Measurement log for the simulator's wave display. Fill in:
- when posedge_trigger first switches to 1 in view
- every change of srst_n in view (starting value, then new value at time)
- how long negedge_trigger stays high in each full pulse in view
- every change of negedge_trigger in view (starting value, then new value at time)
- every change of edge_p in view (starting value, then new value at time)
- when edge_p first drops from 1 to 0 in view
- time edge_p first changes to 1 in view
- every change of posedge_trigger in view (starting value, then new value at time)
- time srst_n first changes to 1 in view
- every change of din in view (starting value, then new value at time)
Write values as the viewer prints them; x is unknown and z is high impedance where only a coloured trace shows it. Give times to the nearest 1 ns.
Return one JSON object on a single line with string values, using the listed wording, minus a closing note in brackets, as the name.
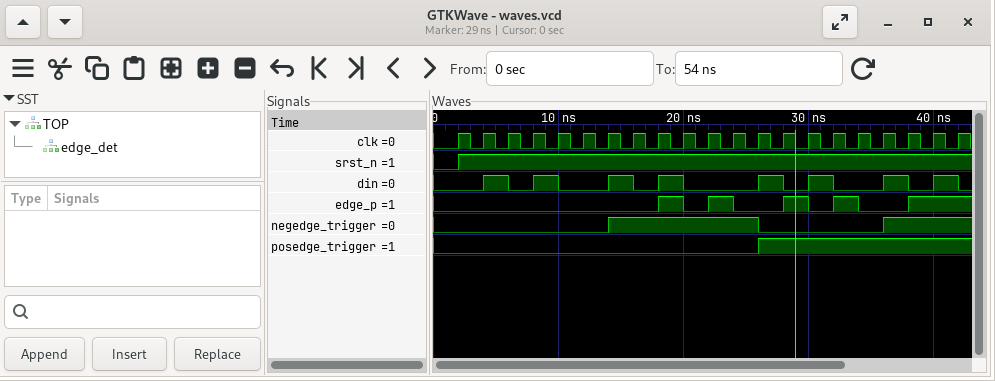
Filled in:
{"when posedge_trigger first switches to 1 in view": "26 ns", "every change of srst_n in view": "0, 1 at 2 ns", "how long negedge_trigger stays high in each full pulse in view": "12 ns", "every change of negedge_trigger in view": "0, 1 at 14 ns, 0 at 26 ns, 1 at 36 ns", "every change of edge_p in view": "0, 1 at 18 ns, 0 at 20 ns, 1 at 22 ns, 0 at 24 ns, 1 at 28 ns, 0 at 30 ns, 1 at 32 ns, 0 at 34 ns, 1 at 38 ns", "when edge_p first drops from 1 to 0 in view": "20 ns", "time edge_p first changes to 1 in view": "18 ns", "every change of posedge_trigger in view": "0, 1 at 26 ns", "time srst_n first changes to 1 in view": "2 ns", "every change of din in view": "0, 1 at 4 ns, 0 at 6 ns, 1 at 8 ns, 0 at 10 ns, 1 at 14 ns, 0 at 16 ns, 1 at 18 ns, 0 at 20 ns, 1 at 26 ns, 0 at 28 ns, 1 at 30 ns, 0 at 32 ns, 1 at 36 ns, 0 at 38 ns, 1 at 40 ns, 0 at 42 ns"}
